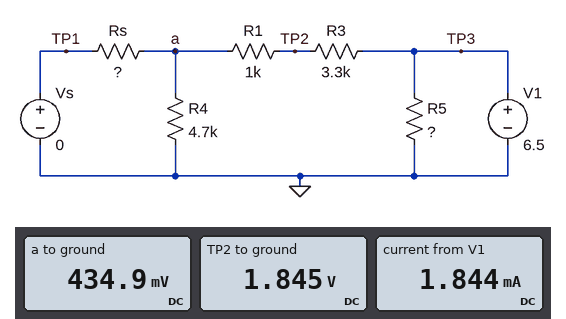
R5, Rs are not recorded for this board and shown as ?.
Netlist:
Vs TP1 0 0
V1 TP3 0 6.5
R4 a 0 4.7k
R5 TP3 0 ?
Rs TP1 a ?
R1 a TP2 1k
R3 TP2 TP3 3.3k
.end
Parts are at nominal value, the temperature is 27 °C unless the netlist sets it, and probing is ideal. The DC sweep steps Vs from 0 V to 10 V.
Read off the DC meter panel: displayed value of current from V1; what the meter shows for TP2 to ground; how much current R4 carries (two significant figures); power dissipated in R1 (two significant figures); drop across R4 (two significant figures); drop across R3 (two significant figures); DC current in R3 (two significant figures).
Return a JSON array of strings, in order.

["1.844 mA", "1.845 V", "93 µA", "2.0 mW", "430 mV", "4.7 V", "1.4 mA"]
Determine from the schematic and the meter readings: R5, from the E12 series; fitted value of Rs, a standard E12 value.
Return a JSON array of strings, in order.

["15 kΩ", "330 Ω"]
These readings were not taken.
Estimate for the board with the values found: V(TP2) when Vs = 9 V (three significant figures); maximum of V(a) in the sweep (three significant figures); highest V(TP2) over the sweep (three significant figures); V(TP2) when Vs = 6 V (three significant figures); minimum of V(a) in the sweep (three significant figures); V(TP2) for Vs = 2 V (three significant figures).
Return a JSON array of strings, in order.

["7.87 V", "9.15 V", "8.54 V", "5.86 V", "435 mV", "3.18 V"]
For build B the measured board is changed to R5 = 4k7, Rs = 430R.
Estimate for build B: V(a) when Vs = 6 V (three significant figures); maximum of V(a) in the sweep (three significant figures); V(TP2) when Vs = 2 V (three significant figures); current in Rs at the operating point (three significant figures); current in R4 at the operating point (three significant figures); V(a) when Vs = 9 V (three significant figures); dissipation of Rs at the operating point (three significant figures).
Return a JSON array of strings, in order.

["5.58 V", "8.94 V", "3.22 V", "1.27 mA", "116 µA", "8.10 V", "692 µW"]
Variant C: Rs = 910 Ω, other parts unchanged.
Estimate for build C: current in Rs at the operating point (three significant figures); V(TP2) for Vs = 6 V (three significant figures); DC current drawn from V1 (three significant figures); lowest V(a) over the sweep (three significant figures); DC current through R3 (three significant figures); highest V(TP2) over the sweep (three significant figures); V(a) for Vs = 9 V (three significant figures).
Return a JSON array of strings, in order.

["1.08 mA", "5.54 V", "1.72 mA", "979 mV", "1.28 mA", "7.72 V", "7.38 V"]
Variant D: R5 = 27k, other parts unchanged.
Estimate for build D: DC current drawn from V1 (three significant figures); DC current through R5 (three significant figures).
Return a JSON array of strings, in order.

["1.65 mA", "241 µA"]
